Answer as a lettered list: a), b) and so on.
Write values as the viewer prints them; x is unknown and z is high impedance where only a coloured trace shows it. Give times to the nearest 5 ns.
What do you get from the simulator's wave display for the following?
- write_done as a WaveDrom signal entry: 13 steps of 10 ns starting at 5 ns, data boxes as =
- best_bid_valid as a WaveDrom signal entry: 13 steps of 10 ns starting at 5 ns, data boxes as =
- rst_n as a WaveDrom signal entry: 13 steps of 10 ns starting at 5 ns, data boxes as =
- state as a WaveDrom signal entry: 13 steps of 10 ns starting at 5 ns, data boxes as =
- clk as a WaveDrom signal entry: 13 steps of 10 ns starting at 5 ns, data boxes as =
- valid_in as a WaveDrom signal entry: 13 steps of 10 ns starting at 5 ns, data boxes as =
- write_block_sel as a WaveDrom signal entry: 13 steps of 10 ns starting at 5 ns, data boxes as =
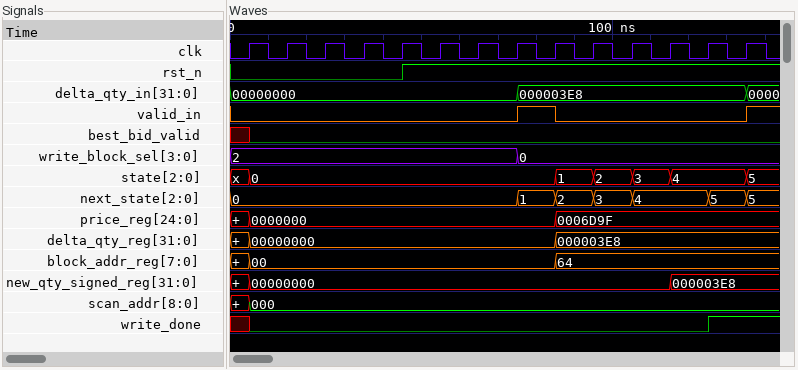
a) {name: 'write_done', wave: '0...........1'}
b) {name: 'best_bid_valid', wave: '0............'}
c) {name: 'rst_n', wave: '0...1........'}
d) {name: 'state', wave: '=.......====.', data: '0 1 2 3 4'}
e) {name: 'clk', wave: 'p............'}
f) {name: 'valid_in', wave: '0......10....'}
g) {name: 'write_block_sel', wave: '=......=.....', data: '2 0'}
